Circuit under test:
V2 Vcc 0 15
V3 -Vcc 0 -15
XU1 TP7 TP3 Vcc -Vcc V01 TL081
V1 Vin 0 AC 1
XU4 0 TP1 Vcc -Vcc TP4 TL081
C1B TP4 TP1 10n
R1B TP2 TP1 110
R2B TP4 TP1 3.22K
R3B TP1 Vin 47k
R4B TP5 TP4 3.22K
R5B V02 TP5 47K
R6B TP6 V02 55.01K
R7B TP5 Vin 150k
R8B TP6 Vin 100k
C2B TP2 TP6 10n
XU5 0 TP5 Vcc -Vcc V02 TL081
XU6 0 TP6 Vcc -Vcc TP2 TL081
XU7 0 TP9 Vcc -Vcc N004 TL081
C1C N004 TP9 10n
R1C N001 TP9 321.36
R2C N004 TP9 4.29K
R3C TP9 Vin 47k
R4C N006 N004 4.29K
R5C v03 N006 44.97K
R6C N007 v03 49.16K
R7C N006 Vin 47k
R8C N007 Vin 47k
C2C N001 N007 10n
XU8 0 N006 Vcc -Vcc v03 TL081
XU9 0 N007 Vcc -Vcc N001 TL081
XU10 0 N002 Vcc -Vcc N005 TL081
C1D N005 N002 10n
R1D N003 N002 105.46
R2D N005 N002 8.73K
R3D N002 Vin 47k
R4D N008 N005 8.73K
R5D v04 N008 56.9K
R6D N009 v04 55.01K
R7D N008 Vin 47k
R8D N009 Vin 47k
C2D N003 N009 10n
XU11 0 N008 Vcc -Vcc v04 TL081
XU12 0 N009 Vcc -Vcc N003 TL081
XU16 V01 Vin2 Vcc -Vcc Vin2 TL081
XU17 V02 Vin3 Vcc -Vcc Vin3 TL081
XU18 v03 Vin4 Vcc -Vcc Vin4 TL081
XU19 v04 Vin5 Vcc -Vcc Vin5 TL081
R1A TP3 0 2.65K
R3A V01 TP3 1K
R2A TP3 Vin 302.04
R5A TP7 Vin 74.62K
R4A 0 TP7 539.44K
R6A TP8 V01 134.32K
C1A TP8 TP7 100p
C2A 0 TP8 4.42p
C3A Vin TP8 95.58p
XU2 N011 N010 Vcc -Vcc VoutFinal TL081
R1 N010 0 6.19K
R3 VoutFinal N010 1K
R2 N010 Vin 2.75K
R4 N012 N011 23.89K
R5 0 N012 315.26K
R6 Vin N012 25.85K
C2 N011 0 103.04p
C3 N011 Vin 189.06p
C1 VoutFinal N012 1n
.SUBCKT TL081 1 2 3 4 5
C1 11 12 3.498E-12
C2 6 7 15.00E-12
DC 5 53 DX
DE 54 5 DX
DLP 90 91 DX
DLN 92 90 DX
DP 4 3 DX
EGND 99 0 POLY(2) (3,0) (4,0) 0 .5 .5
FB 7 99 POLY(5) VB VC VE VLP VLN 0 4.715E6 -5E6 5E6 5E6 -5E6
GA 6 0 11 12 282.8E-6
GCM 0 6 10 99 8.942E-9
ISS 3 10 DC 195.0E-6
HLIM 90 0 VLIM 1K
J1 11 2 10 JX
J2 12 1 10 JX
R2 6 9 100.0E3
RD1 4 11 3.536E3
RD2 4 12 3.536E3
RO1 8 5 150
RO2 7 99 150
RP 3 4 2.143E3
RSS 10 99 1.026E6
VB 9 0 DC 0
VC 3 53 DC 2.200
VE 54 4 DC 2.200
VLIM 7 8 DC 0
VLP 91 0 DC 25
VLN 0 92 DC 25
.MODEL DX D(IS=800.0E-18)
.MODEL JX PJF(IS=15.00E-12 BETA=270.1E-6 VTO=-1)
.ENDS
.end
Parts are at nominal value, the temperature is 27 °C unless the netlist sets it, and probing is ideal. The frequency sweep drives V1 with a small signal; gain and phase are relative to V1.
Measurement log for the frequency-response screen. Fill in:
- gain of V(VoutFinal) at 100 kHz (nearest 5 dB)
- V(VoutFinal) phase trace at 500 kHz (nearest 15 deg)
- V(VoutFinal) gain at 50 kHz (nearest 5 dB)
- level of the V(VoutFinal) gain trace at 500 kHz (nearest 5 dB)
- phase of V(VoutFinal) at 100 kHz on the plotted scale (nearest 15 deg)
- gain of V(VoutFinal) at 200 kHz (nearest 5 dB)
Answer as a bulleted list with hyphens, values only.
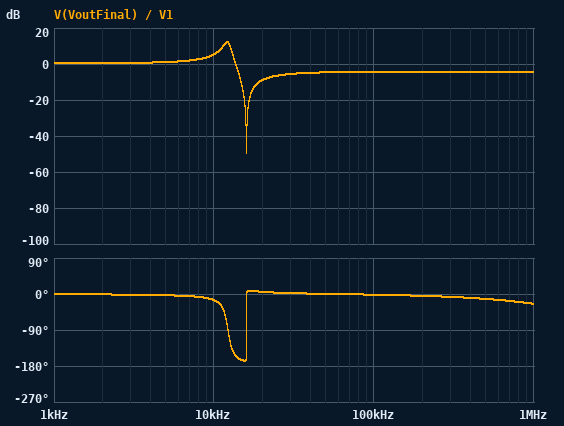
- -5 dB
- -15 deg
- -5 dB
- -5 dB
- 0 deg
- -5 dB
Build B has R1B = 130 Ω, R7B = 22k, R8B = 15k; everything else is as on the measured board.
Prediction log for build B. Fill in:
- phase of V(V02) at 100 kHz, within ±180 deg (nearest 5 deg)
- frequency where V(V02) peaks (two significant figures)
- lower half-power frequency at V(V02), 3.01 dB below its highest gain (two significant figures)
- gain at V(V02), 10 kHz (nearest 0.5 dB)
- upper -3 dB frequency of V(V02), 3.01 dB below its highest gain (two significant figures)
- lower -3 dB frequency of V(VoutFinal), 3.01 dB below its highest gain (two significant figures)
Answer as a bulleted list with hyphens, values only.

- 155 deg
- 22 kHz
- 21 kHz
- 12.0 dB
- 23 kHz
- 11 kHz
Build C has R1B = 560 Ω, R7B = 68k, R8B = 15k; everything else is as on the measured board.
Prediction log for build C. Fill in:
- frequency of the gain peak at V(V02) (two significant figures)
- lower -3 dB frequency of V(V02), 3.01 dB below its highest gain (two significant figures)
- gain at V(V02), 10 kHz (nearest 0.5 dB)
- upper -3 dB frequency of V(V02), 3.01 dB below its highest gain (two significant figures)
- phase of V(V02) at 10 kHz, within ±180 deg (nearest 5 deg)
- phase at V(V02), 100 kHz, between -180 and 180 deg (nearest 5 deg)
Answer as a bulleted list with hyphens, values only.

- 10 kHz
- 7.5 kHz
- 18.0 dB
- 12 kHz
- 110 deg
- 160 deg
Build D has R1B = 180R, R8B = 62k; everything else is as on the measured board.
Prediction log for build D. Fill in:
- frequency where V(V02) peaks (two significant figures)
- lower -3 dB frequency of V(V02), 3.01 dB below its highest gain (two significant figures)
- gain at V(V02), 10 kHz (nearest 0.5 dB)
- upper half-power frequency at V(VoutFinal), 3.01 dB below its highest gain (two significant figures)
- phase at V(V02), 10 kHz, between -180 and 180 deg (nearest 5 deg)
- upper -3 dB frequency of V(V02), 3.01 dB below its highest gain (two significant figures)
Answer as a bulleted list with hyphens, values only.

- 19 kHz
- 17 kHz
- 1.0 dB
- 13 kHz
- 165 deg
- 20 kHz
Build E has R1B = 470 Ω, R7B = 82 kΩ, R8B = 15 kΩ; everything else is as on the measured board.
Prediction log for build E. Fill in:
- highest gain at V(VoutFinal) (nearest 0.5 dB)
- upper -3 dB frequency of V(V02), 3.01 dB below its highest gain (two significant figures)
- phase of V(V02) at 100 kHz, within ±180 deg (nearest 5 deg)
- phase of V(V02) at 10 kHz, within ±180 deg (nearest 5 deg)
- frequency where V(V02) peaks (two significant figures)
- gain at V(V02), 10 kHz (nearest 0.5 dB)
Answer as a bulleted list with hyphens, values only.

- 12.0 dB
- 13 kHz
- 160 deg
- 130 deg
- 11 kHz
- 18.0 dB
